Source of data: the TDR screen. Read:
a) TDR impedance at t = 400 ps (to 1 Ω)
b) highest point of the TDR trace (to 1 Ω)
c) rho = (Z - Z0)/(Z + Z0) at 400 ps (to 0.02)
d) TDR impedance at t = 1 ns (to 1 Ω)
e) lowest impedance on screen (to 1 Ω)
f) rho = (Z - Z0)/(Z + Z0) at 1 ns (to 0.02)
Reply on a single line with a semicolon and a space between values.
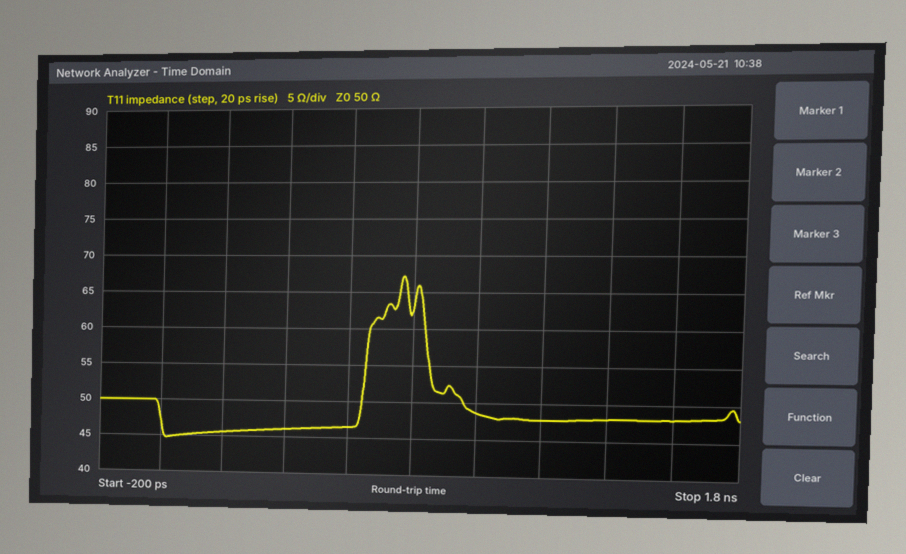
46 Ω; 67 Ω; -0.04; 49 Ω; 45 Ω; -0.02
